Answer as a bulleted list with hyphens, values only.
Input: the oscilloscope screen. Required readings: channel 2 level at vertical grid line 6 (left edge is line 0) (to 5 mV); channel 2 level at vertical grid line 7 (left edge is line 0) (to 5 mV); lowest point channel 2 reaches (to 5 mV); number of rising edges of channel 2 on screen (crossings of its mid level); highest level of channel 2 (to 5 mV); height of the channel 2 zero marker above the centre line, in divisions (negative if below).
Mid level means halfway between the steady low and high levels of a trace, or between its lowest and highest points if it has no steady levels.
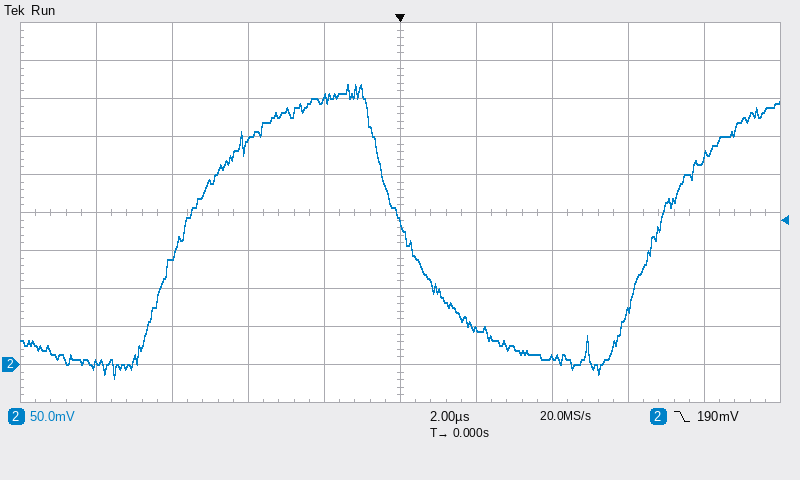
- 45 mV
- 10 mV
- -20 mV
- 2
- 370 mV
- -4.0 div
